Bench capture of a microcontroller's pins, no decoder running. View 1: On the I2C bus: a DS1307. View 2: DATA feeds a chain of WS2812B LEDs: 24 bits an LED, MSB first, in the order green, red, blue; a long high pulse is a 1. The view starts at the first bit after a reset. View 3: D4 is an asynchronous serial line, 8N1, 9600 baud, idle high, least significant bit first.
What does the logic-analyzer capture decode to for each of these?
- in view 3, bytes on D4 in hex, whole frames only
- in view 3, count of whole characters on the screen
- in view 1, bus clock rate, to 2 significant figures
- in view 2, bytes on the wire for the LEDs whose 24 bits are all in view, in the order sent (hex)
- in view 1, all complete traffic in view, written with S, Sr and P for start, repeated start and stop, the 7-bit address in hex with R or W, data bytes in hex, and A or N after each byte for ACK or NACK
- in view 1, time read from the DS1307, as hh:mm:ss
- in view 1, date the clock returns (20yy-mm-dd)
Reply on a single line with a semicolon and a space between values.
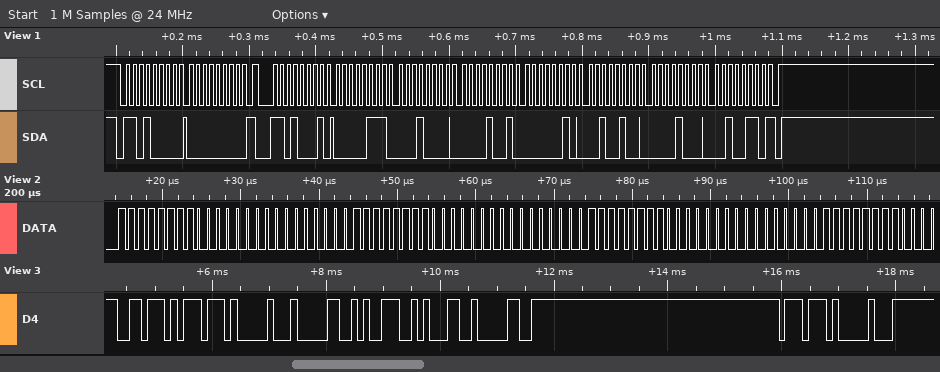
76 77 10 30 39 31 30 77 10; 9; 100 kHz; FF 00 00 FF 00 00 FF 00 00; S 68W A 00 A Sr 68R A 07 A 10 A 09 A 02 A 24 A 08 A 26 N P; 09:10:07; 2026-08-24
